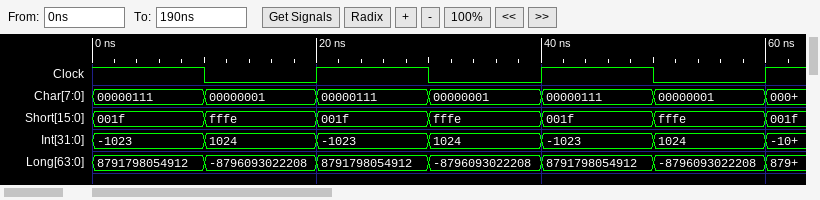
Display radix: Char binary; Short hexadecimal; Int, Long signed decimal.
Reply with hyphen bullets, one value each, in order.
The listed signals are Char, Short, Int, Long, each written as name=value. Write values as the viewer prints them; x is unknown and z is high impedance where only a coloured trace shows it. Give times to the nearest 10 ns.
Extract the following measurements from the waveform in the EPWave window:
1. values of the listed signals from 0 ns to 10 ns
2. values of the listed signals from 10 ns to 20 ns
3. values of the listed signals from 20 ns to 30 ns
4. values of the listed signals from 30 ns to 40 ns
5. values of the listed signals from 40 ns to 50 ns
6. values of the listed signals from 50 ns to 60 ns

- Char=00000111, Short=001f, Int=-1023, Long=8791798054912
- Char=00000001, Short=fffe, Int=1024, Long=-8796093022208
- Char=00000111, Short=001f, Int=-1023, Long=8791798054912
- Char=00000001, Short=fffe, Int=1024, Long=-8796093022208
- Char=00000111, Short=001f, Int=-1023, Long=8791798054912
- Char=00000001, Short=fffe, Int=1024, Long=-8796093022208
